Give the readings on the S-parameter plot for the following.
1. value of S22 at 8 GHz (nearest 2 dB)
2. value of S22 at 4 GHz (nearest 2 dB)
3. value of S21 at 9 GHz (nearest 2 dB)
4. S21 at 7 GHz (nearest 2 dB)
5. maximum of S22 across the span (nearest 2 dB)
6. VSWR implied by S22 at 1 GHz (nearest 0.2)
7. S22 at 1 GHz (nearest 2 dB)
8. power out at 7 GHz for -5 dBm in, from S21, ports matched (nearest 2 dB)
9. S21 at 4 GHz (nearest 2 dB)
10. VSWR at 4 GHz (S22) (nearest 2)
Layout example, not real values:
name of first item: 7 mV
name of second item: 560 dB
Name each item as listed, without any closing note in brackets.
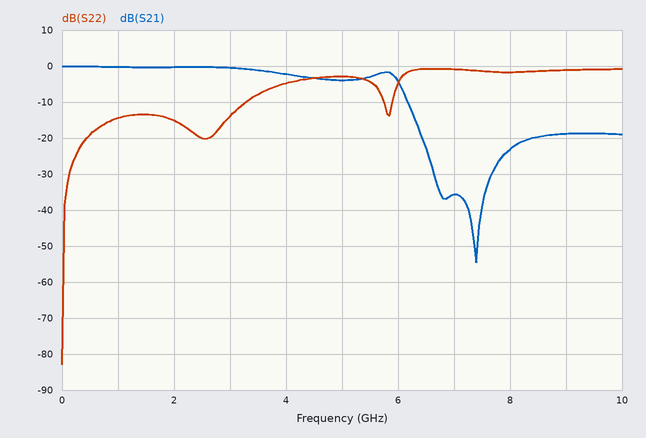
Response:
value of S22 at 8 GHz: -2 dB
value of S22 at 4 GHz: -4 dB
value of S21 at 9 GHz: -18 dB
S21 at 7 GHz: -36 dB
maximum of S22 across the span: 0 dB
VSWR implied by S22 at 1 GHz: 1.4
S22 at 1 GHz: -14 dB
power out at 7 GHz for -5 dBm in, from S21, ports matched: -40 dBm
S21 at 4 GHz: -2 dB
VSWR at 4 GHz (S22): 4
